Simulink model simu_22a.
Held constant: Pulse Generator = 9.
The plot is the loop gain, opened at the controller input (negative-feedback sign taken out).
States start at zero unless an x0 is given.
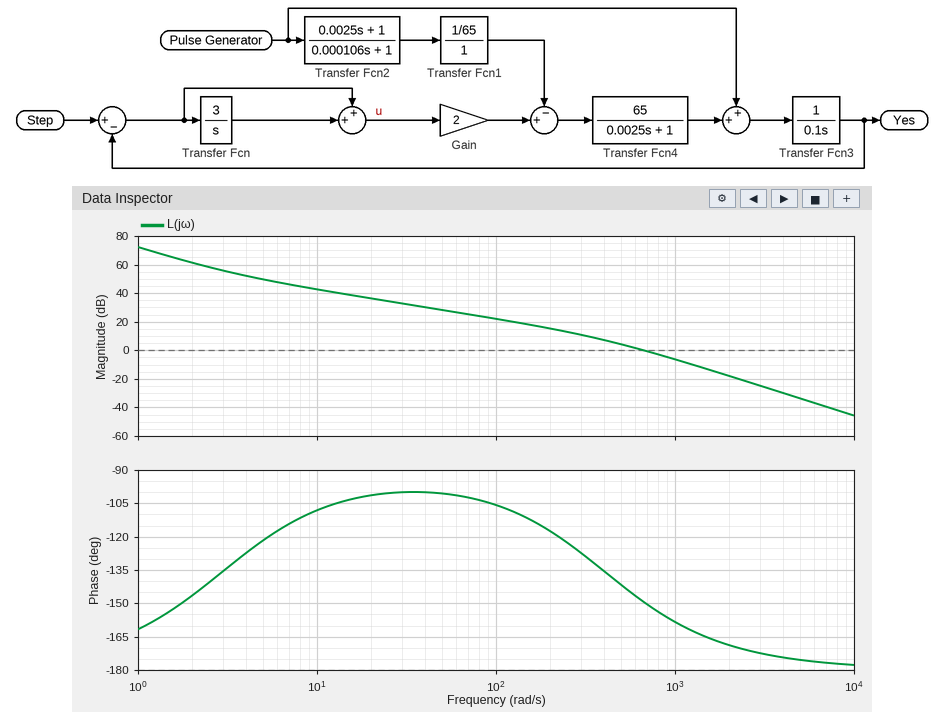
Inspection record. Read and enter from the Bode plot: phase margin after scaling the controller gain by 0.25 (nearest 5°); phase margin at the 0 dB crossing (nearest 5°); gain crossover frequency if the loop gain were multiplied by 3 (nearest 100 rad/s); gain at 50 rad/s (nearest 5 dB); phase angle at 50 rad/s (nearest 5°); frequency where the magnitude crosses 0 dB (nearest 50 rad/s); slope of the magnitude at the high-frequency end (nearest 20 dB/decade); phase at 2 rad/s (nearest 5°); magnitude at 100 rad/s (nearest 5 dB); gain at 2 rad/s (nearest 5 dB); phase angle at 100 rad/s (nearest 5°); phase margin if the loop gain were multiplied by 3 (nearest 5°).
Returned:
55°
30°
1200 rad/s
30 dB
-100°
650 rad/s
-40 dB/decade
-145°
20 dB
60 dB
-105°
20°
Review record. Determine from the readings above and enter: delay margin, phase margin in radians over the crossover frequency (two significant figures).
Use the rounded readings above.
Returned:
0.00081 s
